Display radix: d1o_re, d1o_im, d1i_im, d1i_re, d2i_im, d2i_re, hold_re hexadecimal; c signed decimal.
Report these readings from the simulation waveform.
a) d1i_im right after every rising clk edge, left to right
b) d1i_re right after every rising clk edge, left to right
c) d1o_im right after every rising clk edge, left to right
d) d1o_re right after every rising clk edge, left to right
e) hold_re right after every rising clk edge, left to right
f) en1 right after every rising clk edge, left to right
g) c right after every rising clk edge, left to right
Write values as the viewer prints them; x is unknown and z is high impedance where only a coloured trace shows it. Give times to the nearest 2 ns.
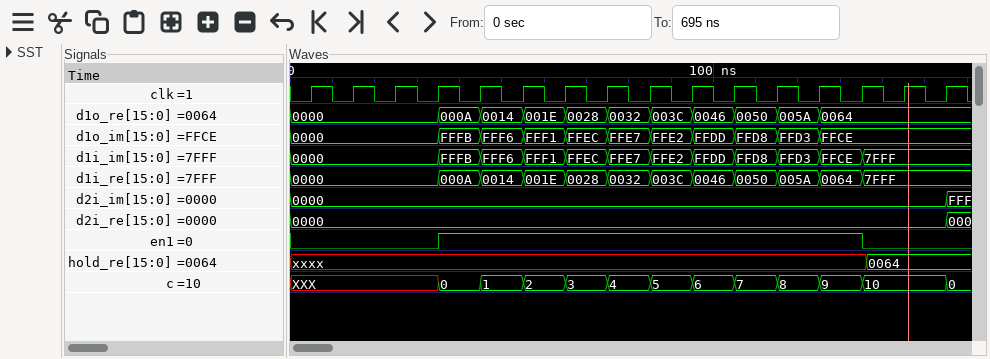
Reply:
0000, 0000, 0000, FFFB, FFF6, FFF1, FFEC, FFE7, FFE2, FFDD, FFD8, FFD3, FFCE, 7FFF, 7FFF, 7FFF
0000, 0000, 0000, 000A, 0014, 001E, 0028, 0032, 003C, 0046, 0050, 005A, 0064, 7FFF, 7FFF, 7FFF
0000, 0000, 0000, FFFB, FFF6, FFF1, FFEC, FFE7, FFE2, FFDD, FFD8, FFD3, FFCE, FFCE, FFCE, FFCE
0000, 0000, 0000, 000A, 0014, 001E, 0028, 0032, 003C, 0046, 0050, 005A, 0064, 0064, 0064, 0064
xxxx, xxxx, xxxx, xxxx, xxxx, xxxx, xxxx, xxxx, xxxx, xxxx, xxxx, xxxx, xxxx, xxxx, 0064, 0064
0 0 0 1 1 1 1 1 1 1 1 1 1 0 0 0
XXX, XXX, XXX, 0, 1, 2, 3, 4, 5, 6, 7, 8, 9, 10, 10, 0
